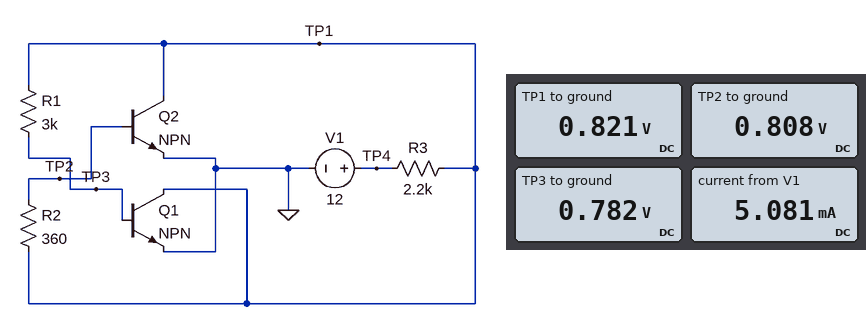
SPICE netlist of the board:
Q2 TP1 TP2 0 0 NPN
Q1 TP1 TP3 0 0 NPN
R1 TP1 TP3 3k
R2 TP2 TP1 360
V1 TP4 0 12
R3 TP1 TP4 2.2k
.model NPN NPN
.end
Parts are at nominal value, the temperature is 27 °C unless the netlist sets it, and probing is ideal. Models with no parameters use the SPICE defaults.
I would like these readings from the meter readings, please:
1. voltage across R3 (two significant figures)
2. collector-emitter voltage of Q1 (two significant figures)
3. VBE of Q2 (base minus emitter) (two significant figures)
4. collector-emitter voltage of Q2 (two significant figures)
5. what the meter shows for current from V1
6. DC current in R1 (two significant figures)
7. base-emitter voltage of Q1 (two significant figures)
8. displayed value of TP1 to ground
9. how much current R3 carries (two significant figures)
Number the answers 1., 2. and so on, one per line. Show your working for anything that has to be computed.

1. 12 V - 821 mV = 11 V
2. 821 mV = 820 mV
3. 808 mV = 810 mV
4. 821 mV = 820 mV
5. 5.081 mA
6. (821 mV - 782 mV) / 3 kΩ = 13 µA
7. 782 mV = 780 mV
8. 0.821 V
9. (12 V - 821 mV) / 2.2 kΩ = 5.1 mA
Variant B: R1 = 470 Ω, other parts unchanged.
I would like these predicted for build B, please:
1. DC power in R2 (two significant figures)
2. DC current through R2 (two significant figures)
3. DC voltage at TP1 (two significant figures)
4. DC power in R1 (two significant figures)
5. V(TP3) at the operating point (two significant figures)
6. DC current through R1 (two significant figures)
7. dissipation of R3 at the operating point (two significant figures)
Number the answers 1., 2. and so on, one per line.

1. 250 nW
2. 26 µA
3. 810 mV
4. 280 nW
5. 800 mV
6. 24 µA
7. 57 mW
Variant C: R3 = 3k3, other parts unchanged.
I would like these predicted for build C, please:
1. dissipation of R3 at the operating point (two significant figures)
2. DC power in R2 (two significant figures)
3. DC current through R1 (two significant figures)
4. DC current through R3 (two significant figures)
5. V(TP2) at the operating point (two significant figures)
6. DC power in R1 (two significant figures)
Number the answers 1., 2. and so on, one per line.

1. 38 mW
2. 200 nW
3. 10 µA
4. 3.4 mA
5. 800 mV
6. 310 nW
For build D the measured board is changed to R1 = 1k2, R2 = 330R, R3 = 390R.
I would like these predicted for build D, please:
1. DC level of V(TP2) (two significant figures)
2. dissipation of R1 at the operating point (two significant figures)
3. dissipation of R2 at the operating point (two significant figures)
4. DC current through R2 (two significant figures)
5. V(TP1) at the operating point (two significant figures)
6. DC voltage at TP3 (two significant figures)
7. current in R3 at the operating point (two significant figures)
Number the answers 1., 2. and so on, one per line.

1. 850 mV
2. 7.1 µW
3. 14 µW
4. 200 µA
5. 920 mV
6. 830 mV
7. 28 mA
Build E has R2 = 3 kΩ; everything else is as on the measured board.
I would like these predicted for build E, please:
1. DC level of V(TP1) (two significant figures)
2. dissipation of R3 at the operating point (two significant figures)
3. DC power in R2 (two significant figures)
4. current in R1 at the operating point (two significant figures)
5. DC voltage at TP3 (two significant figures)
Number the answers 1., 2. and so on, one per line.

1. 870 mV
2. 56 mW
3. 1.9 µW
4. 25 µA
5. 800 mV
